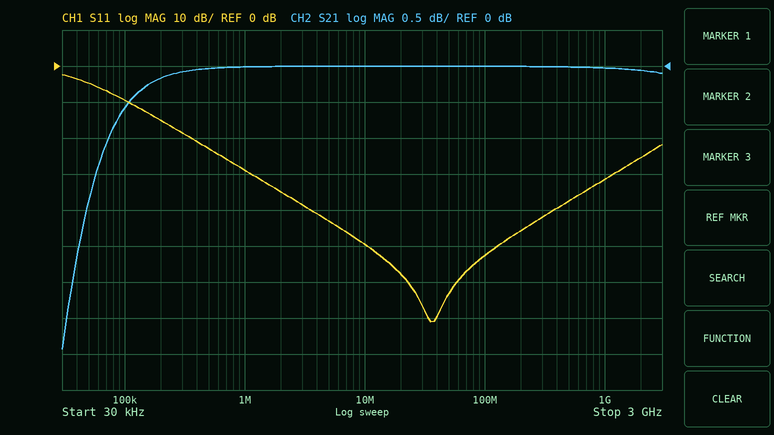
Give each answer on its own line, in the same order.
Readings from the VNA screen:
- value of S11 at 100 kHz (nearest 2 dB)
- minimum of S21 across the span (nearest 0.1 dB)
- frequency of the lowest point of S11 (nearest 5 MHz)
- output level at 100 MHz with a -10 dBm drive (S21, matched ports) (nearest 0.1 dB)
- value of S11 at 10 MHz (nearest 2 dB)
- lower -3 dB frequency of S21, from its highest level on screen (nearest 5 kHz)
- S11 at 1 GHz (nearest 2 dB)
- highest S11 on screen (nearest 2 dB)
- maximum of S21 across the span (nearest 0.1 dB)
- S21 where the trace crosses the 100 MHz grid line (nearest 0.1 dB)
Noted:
-10 dB
-3.9 dB
35 MHz
-10.0 dBm
-50 dB
35 kHz
-32 dB
-2 dB
0.0 dB
0.0 dB
